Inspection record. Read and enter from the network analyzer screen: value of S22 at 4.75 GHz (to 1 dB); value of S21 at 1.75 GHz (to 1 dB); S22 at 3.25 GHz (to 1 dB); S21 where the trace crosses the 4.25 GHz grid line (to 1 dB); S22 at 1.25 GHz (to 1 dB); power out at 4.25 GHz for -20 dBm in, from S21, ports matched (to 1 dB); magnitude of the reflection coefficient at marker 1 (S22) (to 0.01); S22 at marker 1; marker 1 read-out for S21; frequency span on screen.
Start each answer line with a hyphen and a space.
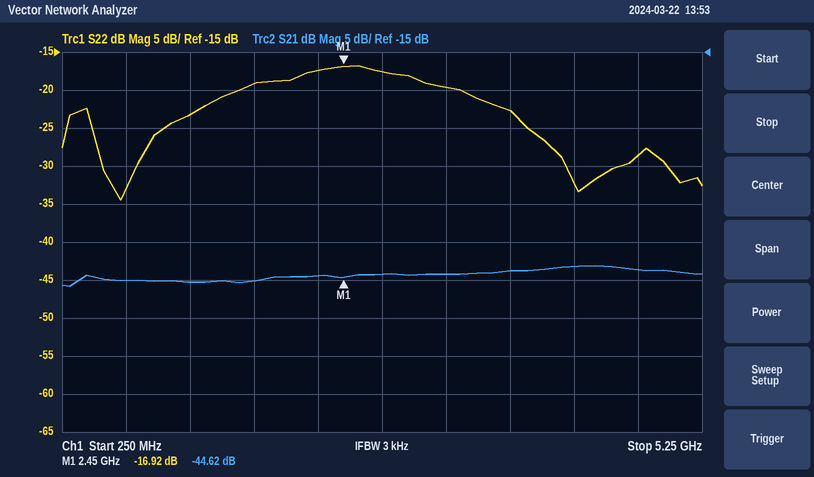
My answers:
- -29 dB
- -45 dB
- -20 dB
- -43 dB
- -23 dB
- -63 dBm
- 0.14
- -16.92 dB
- -44.62 dB
- 5 GHz
